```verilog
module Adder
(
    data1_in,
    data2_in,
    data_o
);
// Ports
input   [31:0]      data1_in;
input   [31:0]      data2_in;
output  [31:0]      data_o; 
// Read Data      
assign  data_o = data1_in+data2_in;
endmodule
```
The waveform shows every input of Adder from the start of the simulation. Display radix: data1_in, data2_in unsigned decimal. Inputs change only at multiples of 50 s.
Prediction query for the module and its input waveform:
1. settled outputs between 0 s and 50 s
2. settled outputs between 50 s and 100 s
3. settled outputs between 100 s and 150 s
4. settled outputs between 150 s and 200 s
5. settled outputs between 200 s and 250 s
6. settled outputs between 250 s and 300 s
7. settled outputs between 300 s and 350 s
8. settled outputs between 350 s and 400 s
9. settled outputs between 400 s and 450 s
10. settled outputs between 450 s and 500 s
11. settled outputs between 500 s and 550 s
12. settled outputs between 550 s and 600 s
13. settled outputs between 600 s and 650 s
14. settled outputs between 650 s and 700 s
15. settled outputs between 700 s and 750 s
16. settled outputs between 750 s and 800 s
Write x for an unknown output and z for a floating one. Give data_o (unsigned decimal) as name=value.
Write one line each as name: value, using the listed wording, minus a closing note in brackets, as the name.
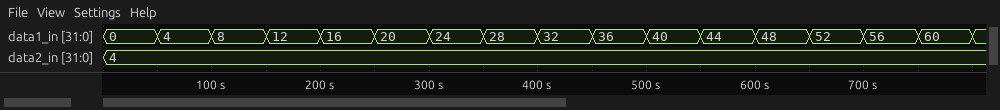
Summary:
settled outputs between 0 s and 50 s: data_o=4
settled outputs between 50 s and 100 s: data_o=8
settled outputs between 100 s and 150 s: data_o=12
settled outputs between 150 s and 200 s: data_o=16
settled outputs between 200 s and 250 s: data_o=20
settled outputs between 250 s and 300 s: data_o=24
settled outputs between 300 s and 350 s: data_o=28
settled outputs between 350 s and 400 s: data_o=32
settled outputs between 400 s and 450 s: data_o=36
settled outputs between 450 s and 500 s: data_o=40
settled outputs between 500 s and 550 s: data_o=44
settled outputs between 550 s and 600 s: data_o=48
settled outputs between 600 s and 650 s: data_o=52
settled outputs between 650 s and 700 s: data_o=56
settled outputs between 700 s and 750 s: data_o=60
settled outputs between 750 s and 800 s: data_o=64
